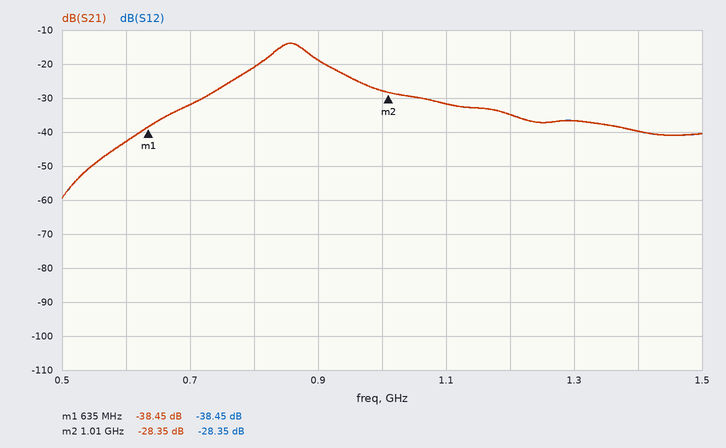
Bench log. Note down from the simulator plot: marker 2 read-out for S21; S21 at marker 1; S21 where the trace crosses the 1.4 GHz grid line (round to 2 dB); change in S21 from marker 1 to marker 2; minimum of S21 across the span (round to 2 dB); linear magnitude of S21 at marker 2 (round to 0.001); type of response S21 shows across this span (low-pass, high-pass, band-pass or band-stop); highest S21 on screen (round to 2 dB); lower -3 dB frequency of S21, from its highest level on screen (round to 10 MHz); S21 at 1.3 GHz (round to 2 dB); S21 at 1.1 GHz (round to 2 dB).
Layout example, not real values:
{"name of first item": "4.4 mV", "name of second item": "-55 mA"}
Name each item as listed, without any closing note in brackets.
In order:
{"marker 2 read-out for S21": "-28.35 dB", "S21 at marker 1": "-38.45 dB", "S21 where the trace crosses the 1.4 GHz grid line": "-40 dB", "change in S21 from marker 1 to marker 2": "10.10 dB", "minimum of S21 across the span": "-60 dB", "linear magnitude of S21 at marker 2": "0.038", "type of response S21 shows across this span": "band-pass", "highest S21 on screen": "-14 dB", "lower -3 dB frequency of S21, from its highest level on screen": "830 MHz", "S21 at 1.3 GHz": "-36 dB", "S21 at 1.1 GHz": "-32 dB"}
